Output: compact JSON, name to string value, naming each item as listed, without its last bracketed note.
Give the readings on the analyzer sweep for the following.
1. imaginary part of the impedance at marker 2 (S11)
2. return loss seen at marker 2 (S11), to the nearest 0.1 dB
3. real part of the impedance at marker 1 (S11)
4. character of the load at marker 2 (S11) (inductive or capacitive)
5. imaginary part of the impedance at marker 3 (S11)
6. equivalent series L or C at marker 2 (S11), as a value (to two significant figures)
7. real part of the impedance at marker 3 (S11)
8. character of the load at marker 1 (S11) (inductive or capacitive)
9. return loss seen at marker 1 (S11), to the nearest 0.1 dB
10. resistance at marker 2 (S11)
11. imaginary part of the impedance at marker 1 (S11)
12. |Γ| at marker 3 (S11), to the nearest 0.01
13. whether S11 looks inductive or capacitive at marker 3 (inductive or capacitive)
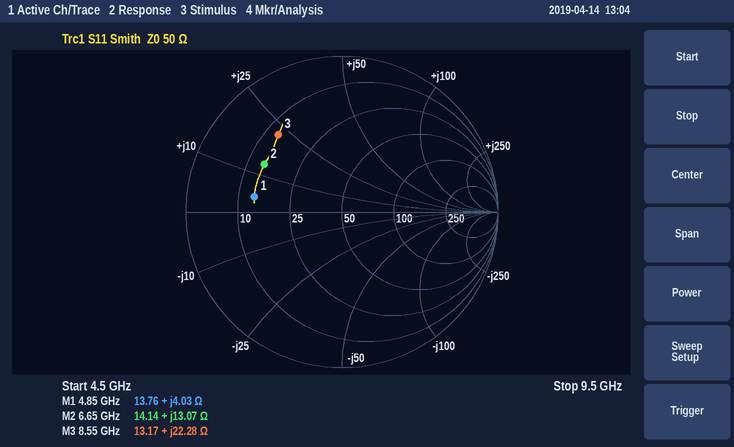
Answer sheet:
{"imaginary part of the impedance at marker 2": "+13.07 Ω", "return loss seen at marker 2 (S11), to the nearest 0.1 dB": "4.7 dB", "real part of the impedance at marker 1": "13.76 Ω", "character of the load at marker 2 (S11)": "inductive", "imaginary part of the impedance at marker 3": "+22.28 Ω", "equivalent series L or C at marker 2 (S11), as a value": "310 pH", "real part of the impedance at marker 3": "13.17 Ω", "character of the load at marker 1 (S11)": "inductive", "return loss seen at marker 1 (S11), to the nearest 0.1 dB": "4.9 dB", "resistance at marker 2": "14.14 Ω", "imaginary part of the impedance at marker 1": "+4.03 Ω", "|Γ| at marker 3 (S11), to the nearest 0.01": "0.64", "whether S11 looks inductive or capacitive at marker 3": "inductive"}
